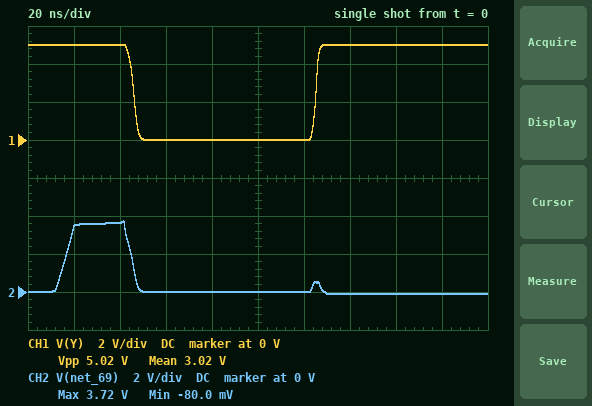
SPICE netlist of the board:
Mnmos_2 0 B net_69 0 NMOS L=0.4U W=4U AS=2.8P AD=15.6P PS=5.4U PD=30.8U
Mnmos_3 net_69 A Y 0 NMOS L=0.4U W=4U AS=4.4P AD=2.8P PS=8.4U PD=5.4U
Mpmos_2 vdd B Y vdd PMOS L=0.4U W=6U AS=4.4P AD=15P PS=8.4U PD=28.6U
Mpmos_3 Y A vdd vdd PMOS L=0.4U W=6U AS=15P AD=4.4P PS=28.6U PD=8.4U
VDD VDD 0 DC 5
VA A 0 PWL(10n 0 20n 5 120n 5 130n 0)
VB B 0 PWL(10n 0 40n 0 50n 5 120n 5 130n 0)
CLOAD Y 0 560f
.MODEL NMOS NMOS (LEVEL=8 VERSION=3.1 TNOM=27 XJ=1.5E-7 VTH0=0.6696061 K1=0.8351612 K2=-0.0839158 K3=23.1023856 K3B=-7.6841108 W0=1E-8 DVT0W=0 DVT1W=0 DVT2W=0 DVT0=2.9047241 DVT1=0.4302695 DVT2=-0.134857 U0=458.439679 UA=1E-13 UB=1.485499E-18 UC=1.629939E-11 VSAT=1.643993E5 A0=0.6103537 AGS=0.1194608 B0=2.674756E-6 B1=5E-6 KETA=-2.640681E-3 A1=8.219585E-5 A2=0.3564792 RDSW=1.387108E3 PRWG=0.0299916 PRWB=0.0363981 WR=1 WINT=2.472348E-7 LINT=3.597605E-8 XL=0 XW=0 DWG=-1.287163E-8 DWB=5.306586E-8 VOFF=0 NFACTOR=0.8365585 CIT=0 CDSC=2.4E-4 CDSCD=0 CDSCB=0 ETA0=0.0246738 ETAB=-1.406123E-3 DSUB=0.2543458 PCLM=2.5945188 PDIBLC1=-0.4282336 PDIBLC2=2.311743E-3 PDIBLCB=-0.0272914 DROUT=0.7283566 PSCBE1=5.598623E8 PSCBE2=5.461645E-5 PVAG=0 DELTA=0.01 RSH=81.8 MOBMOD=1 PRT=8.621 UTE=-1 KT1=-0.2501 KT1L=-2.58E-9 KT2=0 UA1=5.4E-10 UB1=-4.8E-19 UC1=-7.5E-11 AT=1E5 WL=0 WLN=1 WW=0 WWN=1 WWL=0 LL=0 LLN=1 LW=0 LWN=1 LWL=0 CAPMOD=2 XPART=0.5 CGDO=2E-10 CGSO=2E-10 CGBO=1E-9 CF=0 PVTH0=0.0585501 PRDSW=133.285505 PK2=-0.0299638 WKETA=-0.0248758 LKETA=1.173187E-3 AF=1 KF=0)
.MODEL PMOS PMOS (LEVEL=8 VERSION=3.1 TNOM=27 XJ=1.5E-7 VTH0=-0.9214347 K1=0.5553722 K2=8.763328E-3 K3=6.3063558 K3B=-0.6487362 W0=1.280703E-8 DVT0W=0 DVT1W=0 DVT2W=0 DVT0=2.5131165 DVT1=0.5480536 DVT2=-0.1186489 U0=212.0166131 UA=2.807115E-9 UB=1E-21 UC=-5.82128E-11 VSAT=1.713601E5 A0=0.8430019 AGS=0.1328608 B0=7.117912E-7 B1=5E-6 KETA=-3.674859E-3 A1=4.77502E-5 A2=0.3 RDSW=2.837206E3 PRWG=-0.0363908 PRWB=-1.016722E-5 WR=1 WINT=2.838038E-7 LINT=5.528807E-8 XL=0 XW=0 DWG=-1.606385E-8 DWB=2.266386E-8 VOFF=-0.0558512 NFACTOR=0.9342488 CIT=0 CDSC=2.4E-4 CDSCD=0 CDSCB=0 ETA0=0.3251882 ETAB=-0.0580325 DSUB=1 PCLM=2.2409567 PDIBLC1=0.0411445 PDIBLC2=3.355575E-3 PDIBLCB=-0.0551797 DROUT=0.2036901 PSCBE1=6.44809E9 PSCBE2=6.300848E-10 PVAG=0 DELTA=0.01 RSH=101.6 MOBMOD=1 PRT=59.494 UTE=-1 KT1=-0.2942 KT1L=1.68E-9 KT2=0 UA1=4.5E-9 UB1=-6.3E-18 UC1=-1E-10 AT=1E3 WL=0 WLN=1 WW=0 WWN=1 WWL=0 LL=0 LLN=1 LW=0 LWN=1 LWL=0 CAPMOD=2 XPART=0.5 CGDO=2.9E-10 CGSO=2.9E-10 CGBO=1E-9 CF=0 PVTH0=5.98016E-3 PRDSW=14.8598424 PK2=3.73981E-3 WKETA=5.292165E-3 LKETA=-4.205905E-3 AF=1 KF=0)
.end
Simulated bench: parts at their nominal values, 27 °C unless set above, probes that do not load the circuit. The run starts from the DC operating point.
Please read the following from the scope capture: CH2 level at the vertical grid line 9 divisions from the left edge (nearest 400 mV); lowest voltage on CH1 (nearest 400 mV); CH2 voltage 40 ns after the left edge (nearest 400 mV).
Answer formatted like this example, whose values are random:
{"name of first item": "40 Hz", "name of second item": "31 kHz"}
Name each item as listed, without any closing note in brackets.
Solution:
{"CH2 level at the vertical grid line 9 divisions from the left edge": "0 V", "lowest voltage on CH1": "0 V", "CH2 voltage 40 ns after the left edge": "3.6 V"}
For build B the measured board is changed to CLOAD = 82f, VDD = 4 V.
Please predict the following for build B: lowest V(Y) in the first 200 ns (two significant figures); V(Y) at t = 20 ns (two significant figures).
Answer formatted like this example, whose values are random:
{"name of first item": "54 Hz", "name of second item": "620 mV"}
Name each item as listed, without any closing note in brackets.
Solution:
{"lowest V(Y) in the first 200 ns": "-12 mV", "V(Y) at t = 20 ns": "4.0 V"}
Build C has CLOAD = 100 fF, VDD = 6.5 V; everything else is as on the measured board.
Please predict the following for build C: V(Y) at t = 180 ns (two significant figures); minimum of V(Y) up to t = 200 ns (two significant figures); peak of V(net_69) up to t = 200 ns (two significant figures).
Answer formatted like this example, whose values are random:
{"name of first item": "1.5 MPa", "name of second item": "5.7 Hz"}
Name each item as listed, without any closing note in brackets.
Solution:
{"V(Y) at t = 180 ns": "6.5 V", "minimum of V(Y) up to t = 200 ns": "580 mV", "peak of V(net_69) up to t = 200 ns": "3.7 V"}
